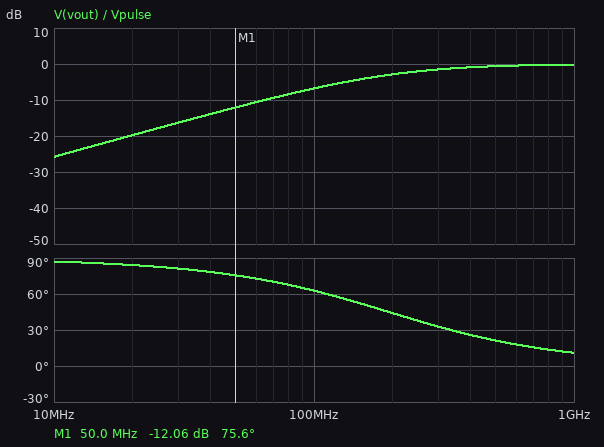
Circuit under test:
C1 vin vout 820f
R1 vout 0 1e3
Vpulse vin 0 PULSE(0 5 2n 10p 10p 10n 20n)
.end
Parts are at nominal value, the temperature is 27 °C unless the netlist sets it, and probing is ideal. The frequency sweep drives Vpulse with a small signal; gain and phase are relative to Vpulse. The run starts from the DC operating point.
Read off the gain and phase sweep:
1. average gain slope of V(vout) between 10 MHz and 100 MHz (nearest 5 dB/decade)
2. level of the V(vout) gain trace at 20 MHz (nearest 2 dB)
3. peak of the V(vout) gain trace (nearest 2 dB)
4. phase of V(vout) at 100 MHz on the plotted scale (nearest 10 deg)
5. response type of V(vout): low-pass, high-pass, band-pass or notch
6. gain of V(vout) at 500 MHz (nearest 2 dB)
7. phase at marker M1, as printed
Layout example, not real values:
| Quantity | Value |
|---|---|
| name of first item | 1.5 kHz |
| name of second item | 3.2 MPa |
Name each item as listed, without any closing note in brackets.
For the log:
| Quantity | Value |
|---|---|
| average gain slope of V(vout) between 10 MHz and 100 MHz | 20 dB/decade |
| level of the V(vout) gain trace at 20 MHz | -20 dB |
| peak of the V(vout) gain trace | 0 dB |
| phase of V(vout) at 100 MHz on the plotted scale | 60 deg |
| response type of V(vout): low-pass, high-pass, band-pass or notch | high-pass |
| gain of V(vout) at 500 MHz | 0 dB |
| phase at marker M1, as printed | 75.6 deg |
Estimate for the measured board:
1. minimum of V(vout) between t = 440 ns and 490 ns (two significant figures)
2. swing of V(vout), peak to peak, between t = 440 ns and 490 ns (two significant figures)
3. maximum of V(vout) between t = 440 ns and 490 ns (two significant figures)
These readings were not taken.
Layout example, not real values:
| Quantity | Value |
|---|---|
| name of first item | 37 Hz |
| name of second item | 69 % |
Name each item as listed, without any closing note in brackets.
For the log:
| Quantity | Value |
|---|---|
| minimum of V(vout) between t = 440 ns and 490 ns | -5.0 V |
| swing of V(vout), peak to peak, between t = 440 ns and 490 ns | 9.9 V |
| maximum of V(vout) between t = 440 ns and 490 ns | 5.0 V |
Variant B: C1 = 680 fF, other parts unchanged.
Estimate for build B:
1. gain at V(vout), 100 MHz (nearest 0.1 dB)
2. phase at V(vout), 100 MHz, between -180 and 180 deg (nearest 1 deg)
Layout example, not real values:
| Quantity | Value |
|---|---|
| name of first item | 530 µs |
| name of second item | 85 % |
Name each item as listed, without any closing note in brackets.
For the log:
| Quantity | Value |
|---|---|
| gain at V(vout), 100 MHz | -8.1 dB |
| phase at V(vout), 100 MHz, between -180 and 180 deg | 67 deg |
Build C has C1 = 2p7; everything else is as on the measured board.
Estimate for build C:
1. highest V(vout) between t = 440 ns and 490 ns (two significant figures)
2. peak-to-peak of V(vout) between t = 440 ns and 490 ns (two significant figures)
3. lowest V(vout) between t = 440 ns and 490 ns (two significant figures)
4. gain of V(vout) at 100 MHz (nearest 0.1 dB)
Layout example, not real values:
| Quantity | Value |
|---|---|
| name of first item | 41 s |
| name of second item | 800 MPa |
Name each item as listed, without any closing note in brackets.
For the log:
| Quantity | Value |
|---|---|
| highest V(vout) between t = 440 ns and 490 ns | 4.9 V |
| peak-to-peak of V(vout) between t = 440 ns and 490 ns | 9.7 V |
| lowest V(vout) between t = 440 ns and 490 ns | -4.9 V |
| gain of V(vout) at 100 MHz | -1.3 dB |
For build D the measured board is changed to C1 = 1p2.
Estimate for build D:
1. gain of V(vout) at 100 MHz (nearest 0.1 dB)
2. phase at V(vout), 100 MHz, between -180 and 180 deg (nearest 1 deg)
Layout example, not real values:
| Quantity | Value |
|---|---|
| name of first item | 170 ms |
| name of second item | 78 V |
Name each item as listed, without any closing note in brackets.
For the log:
| Quantity | Value |
|---|---|
| gain of V(vout) at 100 MHz | -4.4 dB |
| phase at V(vout), 100 MHz, between -180 and 180 deg | 53 deg |
